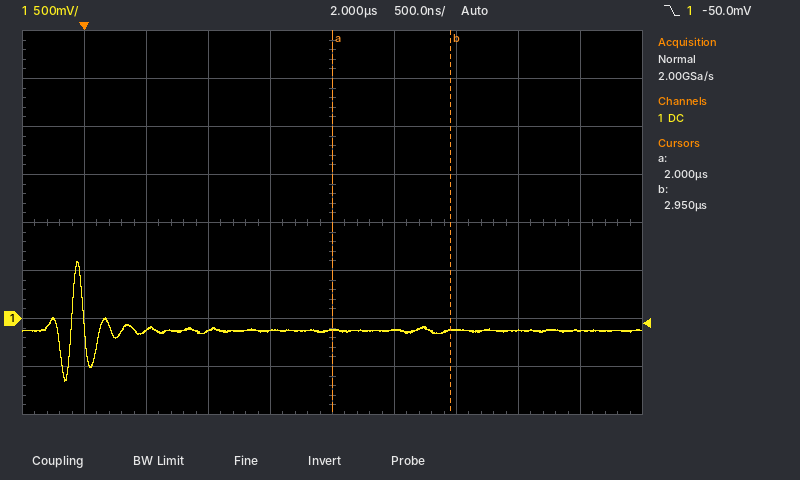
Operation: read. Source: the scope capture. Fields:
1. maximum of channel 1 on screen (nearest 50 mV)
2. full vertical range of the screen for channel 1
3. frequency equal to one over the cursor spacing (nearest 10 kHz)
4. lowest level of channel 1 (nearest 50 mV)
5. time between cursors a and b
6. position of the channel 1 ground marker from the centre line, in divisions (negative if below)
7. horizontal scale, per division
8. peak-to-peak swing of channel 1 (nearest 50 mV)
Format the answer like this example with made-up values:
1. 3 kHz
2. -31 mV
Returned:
1. 600 mV
2. 4 V
3. 1.05 MHz
4. -650 mV
5. 950 ns
6. -2.0 div
7. 500 ns
8. 1.25 V
